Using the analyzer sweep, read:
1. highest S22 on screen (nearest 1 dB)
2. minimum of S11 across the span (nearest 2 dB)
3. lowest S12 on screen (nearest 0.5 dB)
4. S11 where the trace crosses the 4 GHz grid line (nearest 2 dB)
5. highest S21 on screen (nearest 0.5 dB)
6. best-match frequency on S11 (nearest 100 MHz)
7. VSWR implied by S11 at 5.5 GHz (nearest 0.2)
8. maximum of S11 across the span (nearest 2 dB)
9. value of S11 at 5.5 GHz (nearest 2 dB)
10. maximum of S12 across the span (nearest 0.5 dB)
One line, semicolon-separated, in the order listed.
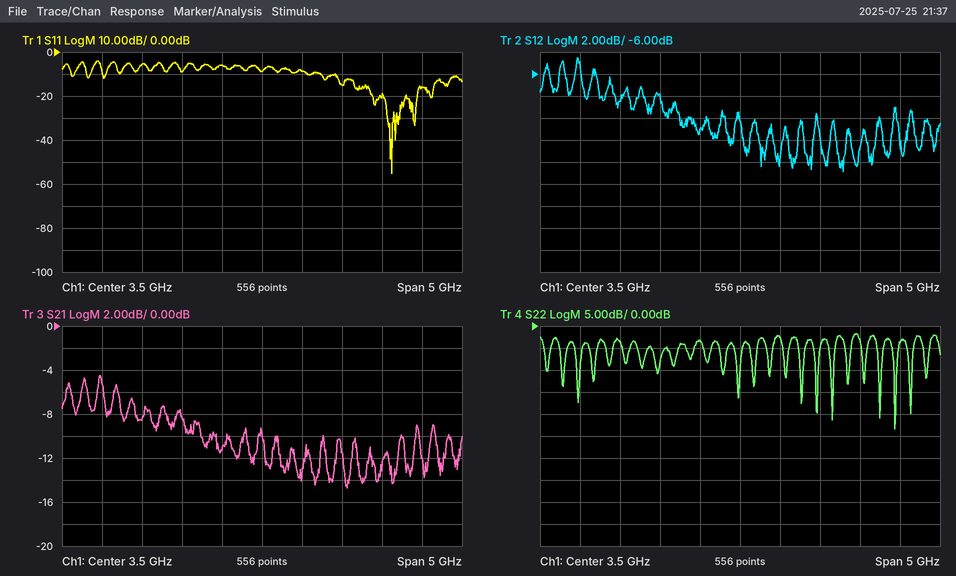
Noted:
-2 dB; -56 dB; -15.0 dB; -8 dB; -4.5 dB; 5.1 GHz; 1.4; -4 dB; -16 dB; -4.5 dB
